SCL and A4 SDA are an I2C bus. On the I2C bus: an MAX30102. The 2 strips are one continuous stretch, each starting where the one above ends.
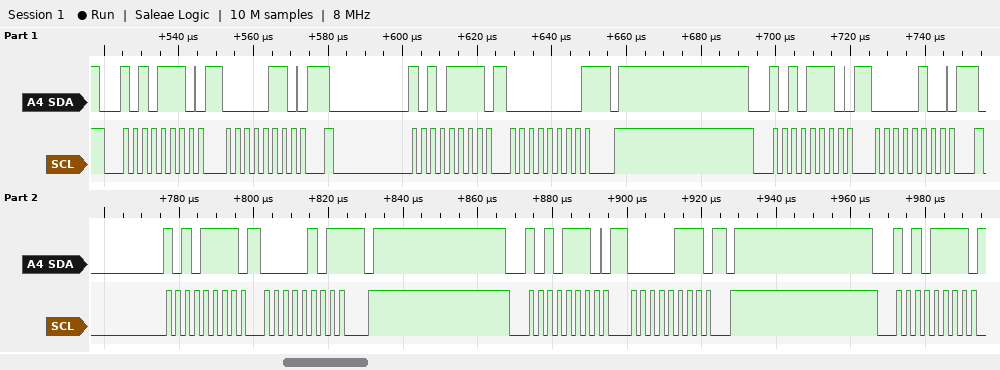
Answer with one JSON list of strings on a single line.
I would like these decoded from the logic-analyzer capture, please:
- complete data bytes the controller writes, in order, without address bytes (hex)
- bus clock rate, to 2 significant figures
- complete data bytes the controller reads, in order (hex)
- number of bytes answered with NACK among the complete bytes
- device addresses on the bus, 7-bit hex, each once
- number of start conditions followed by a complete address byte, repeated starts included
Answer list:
["06 04 07", "400 kHz", "00 05", "2", "0x57", "6"]
